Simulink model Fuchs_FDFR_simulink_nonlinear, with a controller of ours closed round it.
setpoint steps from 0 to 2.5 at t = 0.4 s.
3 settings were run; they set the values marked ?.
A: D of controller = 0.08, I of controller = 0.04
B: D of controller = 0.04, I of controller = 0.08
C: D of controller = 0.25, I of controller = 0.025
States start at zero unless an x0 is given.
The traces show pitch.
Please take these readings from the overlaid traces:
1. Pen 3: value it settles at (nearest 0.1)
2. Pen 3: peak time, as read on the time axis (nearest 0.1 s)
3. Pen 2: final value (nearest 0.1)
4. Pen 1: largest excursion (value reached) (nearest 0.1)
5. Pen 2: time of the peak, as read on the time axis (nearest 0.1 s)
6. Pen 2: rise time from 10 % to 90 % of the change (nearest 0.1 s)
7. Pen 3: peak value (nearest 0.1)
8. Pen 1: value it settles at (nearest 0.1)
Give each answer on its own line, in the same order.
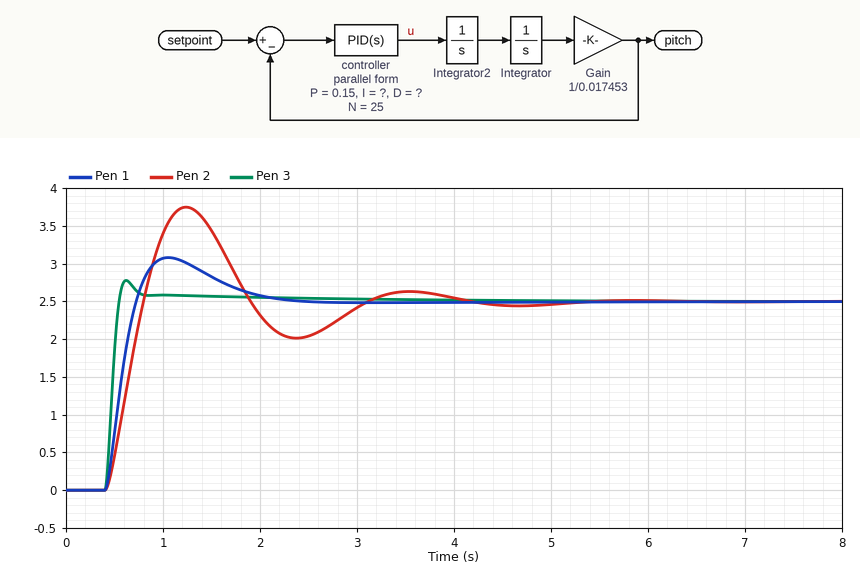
2.5
0.6 s
2.5
3.1
1.2 s
0.3 s
2.8
2.5
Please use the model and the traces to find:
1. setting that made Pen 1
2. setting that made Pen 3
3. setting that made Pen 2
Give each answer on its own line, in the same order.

A
C
B
